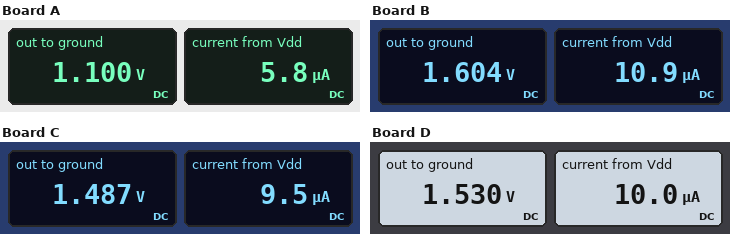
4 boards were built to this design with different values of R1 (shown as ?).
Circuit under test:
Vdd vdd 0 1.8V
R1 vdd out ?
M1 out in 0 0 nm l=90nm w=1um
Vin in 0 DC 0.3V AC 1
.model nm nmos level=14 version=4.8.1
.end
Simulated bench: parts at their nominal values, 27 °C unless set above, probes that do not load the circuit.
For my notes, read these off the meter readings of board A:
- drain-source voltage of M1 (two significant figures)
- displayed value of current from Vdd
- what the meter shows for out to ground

1.1 V
5.8 µA
1.100 V
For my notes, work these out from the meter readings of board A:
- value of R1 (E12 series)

120 kΩ
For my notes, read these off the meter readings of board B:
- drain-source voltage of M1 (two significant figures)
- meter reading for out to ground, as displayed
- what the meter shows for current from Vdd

1.6 V
1.604 V
10.9 µA
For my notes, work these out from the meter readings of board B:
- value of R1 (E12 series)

18 kΩ
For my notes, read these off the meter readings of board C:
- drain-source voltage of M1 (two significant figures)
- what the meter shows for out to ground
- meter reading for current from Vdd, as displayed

1.5 V
1.487 V
9.5 µA
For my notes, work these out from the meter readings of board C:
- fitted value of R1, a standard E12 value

33 kΩ
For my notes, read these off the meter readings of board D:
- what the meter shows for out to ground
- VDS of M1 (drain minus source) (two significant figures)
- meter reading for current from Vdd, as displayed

1.530 V
1.5 V
10.0 µA
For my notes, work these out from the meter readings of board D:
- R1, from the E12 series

27 kΩ
